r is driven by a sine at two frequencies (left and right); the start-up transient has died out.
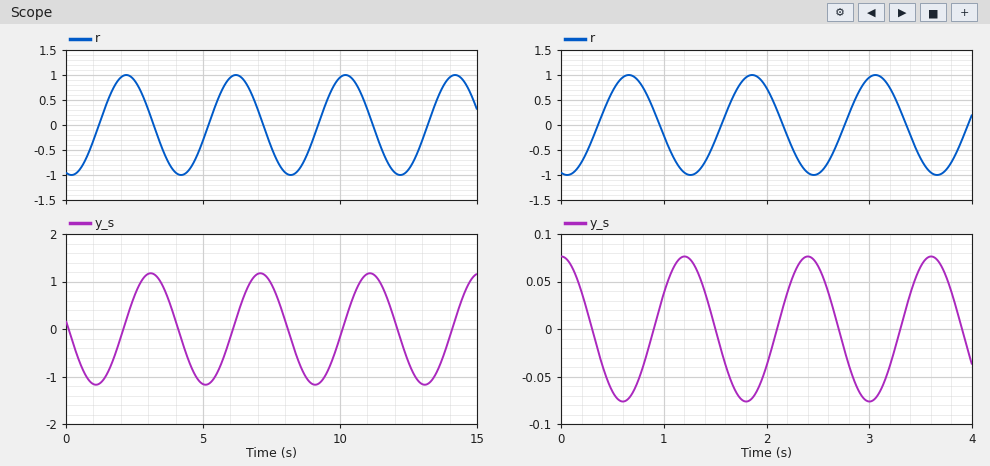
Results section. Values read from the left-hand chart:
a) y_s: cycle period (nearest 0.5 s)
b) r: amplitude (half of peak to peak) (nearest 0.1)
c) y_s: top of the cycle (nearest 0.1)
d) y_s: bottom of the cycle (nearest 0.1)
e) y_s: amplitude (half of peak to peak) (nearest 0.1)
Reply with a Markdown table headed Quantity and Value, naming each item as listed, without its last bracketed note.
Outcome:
| Quantity | Value |
|---|---|
| y_s: cycle period | 4.0 s |
| r: amplitude (half of peak to peak) | 1.0 |
| y_s: top of the cycle | 1.2 |
| y_s: bottom of the cycle | -1.2 |
| y_s: amplitude (half of peak to peak) | 1.2 |
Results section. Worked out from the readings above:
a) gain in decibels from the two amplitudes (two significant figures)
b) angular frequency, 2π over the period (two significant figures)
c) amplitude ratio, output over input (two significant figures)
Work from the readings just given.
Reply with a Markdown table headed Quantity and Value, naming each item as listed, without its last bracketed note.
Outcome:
| Quantity | Value |
|---|---|
| gain in decibels from the two amplitudes | 1.6 dB |
| angular frequency, 2π over the period | 1.6 rad/s |
| amplitude ratio, output over input | 1.2 |
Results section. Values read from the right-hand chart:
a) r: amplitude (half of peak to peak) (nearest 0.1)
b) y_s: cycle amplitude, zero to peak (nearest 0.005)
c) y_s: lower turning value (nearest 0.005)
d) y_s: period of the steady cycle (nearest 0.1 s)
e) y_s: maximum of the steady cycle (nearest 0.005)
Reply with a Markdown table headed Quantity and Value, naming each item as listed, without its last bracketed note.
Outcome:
| Quantity | Value |
|---|---|
| r: amplitude (half of peak to peak) | 1.0 |
| y_s: cycle amplitude, zero to peak | 0.075 |
| y_s: lower turning value | -0.075 |
| y_s: period of the steady cycle | 1.2 s |
| y_s: maximum of the steady cycle | 0.075 |
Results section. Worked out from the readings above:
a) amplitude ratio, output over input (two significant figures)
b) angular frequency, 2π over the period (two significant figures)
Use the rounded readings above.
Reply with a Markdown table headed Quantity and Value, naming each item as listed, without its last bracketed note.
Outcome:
| Quantity | Value |
|---|---|
| amplitude ratio, output over input | 0.075 |
| angular frequency, 2π over the period | 5.2 rad/s |
